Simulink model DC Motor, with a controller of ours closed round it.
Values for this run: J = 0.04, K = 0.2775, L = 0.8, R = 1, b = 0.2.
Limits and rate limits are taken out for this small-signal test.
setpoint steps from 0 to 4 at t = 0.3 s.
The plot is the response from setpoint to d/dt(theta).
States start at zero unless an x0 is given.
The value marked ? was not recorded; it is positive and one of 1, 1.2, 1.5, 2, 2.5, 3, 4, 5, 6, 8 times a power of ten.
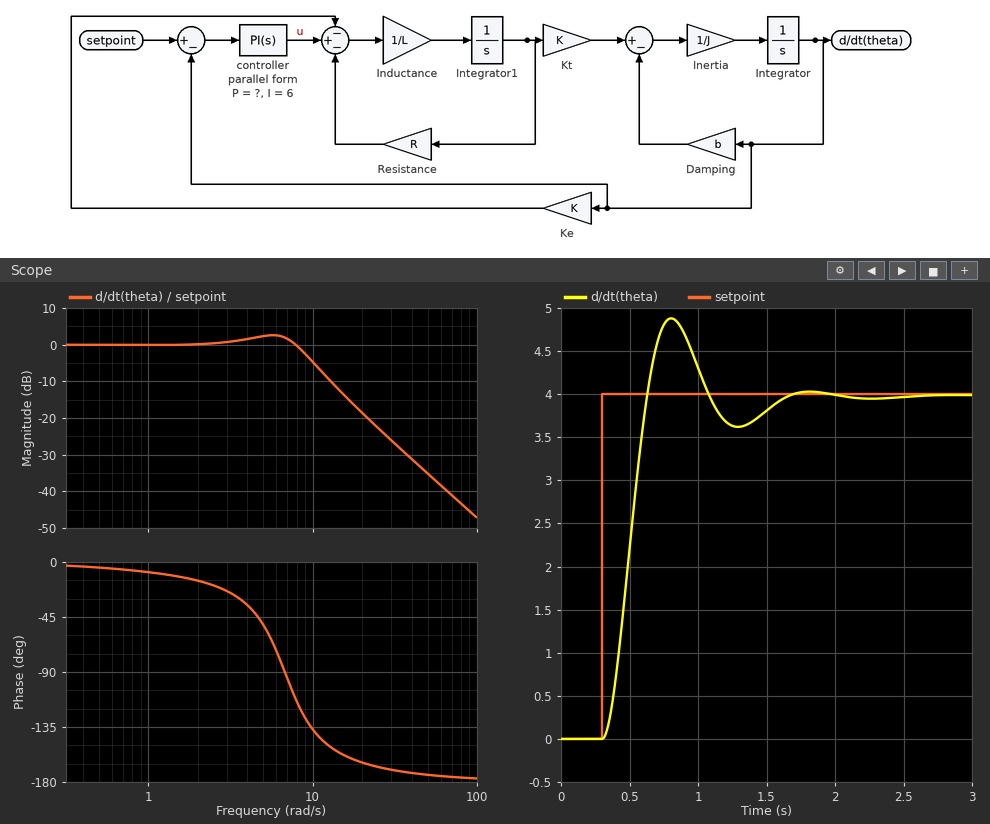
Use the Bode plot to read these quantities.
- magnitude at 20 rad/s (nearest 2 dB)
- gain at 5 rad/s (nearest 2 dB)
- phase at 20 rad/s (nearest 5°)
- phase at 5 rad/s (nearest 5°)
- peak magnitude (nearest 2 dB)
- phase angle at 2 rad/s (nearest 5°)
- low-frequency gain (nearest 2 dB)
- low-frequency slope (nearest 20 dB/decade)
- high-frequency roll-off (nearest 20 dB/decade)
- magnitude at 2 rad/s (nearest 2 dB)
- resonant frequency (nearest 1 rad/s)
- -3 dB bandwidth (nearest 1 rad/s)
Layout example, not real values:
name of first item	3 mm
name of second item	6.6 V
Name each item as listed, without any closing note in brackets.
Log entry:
magnitude at 20 rad/s	-18 dB
gain at 5 rad/s	2 dB
phase at 20 rad/s	-165°
phase at 5 rad/s	-50°
peak magnitude	2 dB
phase angle at 2 rad/s	-15°
low-frequency gain	0 dB
low-frequency slope	0 dB/decade
high-frequency roll-off	-40 dB/decade
magnitude at 2 rad/s	0 dB
resonant frequency	6 rad/s
-3 dB bandwidth	9 rad/s
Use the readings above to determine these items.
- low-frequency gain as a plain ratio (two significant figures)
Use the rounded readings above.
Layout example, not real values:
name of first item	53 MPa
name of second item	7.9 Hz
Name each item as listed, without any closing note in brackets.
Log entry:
low-frequency gain as a plain ratio	1.0
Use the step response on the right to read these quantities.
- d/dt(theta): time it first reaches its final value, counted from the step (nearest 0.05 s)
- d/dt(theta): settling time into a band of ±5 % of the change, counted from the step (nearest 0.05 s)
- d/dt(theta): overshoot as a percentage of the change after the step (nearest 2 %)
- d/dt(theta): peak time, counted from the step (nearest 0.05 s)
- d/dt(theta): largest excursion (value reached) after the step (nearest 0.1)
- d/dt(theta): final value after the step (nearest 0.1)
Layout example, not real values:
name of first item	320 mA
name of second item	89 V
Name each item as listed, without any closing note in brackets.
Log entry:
d/dt(theta): time it first reaches its final value, counted from the step	0.35 s
d/dt(theta): settling time into a band of ±5 % of the change, counted from the step	1.20 s
d/dt(theta): overshoot as a percentage of the change after the step	22 %
d/dt(theta): peak time, counted from the step	0.50 s
d/dt(theta): largest excursion (value reached) after the step	4.9
d/dt(theta): final value after the step	4.0
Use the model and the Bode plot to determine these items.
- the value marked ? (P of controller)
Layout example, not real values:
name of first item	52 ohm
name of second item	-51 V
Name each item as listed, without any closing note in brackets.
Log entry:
the value marked ?	5
